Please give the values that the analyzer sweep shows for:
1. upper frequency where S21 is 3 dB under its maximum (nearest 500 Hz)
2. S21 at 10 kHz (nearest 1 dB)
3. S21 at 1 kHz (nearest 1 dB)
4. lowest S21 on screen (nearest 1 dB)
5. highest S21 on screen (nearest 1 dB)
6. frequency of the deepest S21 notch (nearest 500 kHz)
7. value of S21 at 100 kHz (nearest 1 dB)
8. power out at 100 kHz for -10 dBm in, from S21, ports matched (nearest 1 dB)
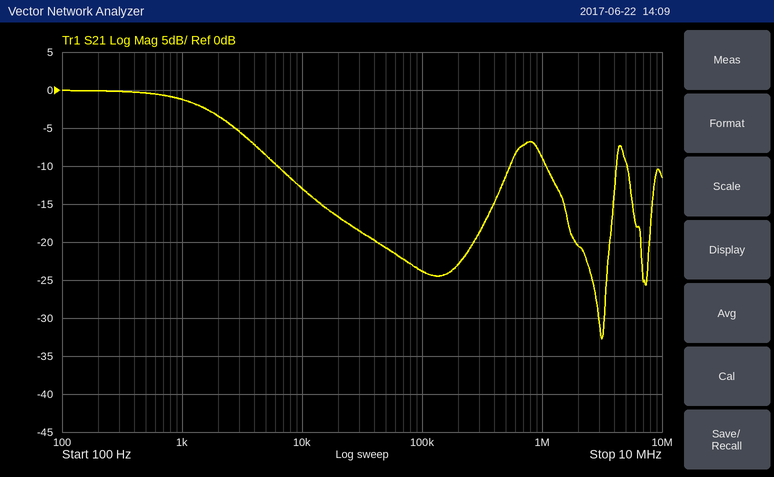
2.0 kHz
-13 dB
-1 dB
-33 dB
0 dB
3.0 MHz
-24 dB
-34 dBm
